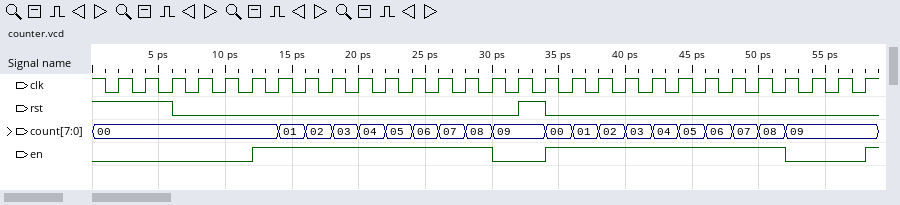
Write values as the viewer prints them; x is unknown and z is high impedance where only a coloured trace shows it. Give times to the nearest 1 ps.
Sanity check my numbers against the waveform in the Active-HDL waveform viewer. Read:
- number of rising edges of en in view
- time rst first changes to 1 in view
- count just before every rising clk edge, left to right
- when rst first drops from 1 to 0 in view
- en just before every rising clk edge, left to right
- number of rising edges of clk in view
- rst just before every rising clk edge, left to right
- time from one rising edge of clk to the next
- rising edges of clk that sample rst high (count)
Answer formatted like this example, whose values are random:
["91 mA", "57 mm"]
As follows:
["3", "32 ps", "00, 00, 00, 00, 00, 00, 00, 01, 02, 03, 04, 05, 06, 07, 08, 09, 09, 00, 01, 02, 03, 04, 05, 06, 07, 08, 09, 09, 09", "6 ps", "0 0 0 0 0 0 1 1 1 1 1 1 1 1 1 0 0 1 1 1 1 1 1 1 1 1 0 0 0", "29", "1 1 1 0 0 0 0 0 0 0 0 0 0 0 0 0 1 0 0 0 0 0 0 0 0 0 0 0 0", "2 ps", "4"]
